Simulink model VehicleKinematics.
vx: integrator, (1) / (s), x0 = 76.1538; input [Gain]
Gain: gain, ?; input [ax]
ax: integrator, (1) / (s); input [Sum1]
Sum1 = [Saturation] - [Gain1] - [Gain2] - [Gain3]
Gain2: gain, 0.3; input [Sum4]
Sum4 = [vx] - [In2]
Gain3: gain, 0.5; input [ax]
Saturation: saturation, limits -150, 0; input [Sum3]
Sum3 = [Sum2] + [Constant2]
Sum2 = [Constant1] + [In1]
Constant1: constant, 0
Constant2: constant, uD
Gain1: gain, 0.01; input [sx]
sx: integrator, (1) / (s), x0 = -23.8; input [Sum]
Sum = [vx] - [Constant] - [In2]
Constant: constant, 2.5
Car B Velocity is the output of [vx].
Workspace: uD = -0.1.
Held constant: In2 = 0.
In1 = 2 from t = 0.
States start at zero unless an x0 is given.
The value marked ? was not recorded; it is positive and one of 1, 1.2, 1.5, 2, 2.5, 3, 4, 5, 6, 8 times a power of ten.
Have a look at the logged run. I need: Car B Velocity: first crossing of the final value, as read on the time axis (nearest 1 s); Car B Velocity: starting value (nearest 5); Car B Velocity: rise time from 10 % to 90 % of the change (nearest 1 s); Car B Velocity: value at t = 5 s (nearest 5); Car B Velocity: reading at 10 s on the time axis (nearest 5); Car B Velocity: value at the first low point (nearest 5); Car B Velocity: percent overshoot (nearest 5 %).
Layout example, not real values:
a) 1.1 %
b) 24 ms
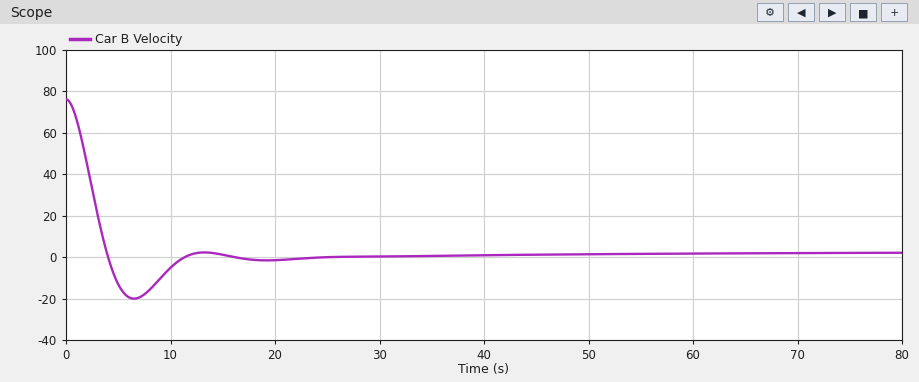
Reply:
a) 4 s
b) 75
c) 3 s
d) -15
e) -5
f) -20
g) 30 %
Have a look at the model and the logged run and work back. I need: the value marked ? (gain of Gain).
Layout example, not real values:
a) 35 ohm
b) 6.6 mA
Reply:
a) 1
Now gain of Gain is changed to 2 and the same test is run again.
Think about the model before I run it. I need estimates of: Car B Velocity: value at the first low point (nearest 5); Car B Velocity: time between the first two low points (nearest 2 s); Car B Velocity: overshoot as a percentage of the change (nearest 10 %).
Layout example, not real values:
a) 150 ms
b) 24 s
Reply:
a) -30
b) 8 s
c) 40 %
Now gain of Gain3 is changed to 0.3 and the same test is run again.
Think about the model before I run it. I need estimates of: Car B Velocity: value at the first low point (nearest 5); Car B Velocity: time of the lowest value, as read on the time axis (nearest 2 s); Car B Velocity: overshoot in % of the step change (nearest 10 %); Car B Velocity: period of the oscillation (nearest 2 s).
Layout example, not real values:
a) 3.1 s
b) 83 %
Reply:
a) -35
b) 6 s
c) 50 %
d) 12 s
